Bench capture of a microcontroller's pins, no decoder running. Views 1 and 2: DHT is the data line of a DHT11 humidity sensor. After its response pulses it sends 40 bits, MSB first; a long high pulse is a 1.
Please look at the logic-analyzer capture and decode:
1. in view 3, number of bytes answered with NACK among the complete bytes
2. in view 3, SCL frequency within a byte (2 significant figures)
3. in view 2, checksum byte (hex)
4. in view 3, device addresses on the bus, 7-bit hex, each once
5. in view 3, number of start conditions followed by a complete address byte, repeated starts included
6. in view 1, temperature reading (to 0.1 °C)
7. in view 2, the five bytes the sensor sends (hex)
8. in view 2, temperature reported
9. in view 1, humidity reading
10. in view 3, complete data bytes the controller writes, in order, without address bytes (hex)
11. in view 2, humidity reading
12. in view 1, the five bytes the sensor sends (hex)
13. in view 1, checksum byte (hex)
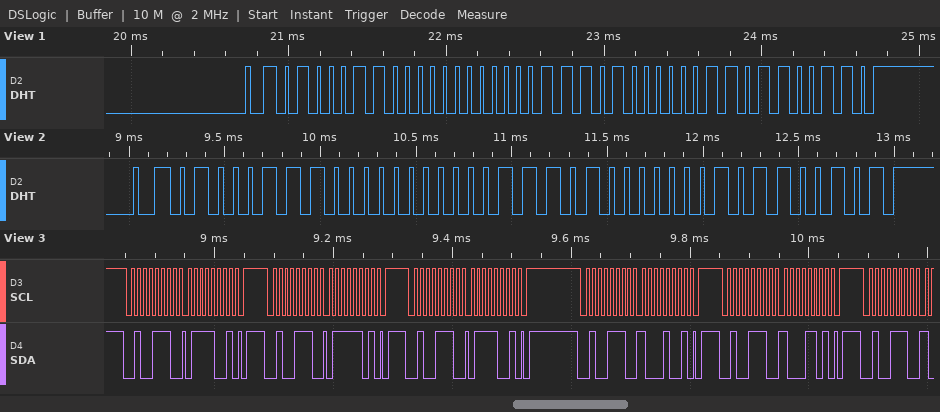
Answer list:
0
100 kHz
0x65
0x27
6
29.3 °C
47 00 1D 01 65
29.1 °C
70 %
79 7D 79 89 8D
71 %
46 00 1D 03 66
0x66
